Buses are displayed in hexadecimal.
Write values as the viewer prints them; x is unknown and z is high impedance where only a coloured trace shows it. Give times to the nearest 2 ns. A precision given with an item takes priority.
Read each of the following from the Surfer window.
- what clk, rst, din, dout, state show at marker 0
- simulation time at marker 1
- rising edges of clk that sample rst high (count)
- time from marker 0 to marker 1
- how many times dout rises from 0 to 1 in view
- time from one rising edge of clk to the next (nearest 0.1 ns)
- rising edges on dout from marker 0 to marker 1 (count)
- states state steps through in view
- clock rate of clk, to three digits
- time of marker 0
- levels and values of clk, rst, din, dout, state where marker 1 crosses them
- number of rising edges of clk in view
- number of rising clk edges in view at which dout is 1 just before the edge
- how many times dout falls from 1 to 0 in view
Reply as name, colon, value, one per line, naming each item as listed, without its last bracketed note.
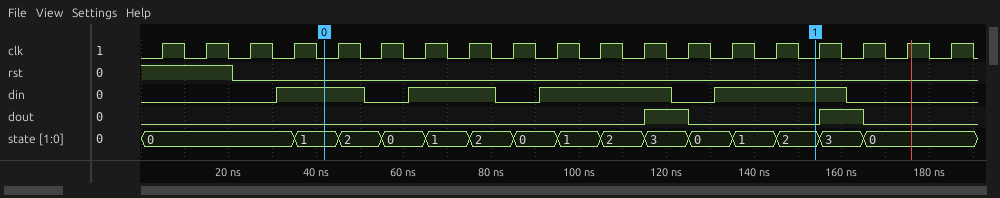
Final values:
what clk, rst, din, dout, state show at marker 0: clk=0, rst=0, din=1, dout=0, state=1
simulation time at marker 1: 154 ns
rising edges of clk that sample rst high: 2
time from marker 0 to marker 1: 112 ns
how many times dout rises from 0 to 1 in view: 2
time from one rising edge of clk to the next: 10 ns
rising edges on dout from marker 0 to marker 1: 1
states state steps through in view: 0, 1, 2, 0, 1, 2, 0, 1, 2, 3, 0, 1, 2, 3, 0
clock rate of clk, to three digits: 100 MHz
time of marker 0: 42 ns
levels and values of clk, rst, din, dout, state where marker 1 crosses them: clk=0, rst=0, din=1, dout=0, state=2
number of rising edges of clk in view: 19
number of rising clk edges in view at which dout is 1 just before the edge: 2
how many times dout falls from 1 to 0 in view: 2
